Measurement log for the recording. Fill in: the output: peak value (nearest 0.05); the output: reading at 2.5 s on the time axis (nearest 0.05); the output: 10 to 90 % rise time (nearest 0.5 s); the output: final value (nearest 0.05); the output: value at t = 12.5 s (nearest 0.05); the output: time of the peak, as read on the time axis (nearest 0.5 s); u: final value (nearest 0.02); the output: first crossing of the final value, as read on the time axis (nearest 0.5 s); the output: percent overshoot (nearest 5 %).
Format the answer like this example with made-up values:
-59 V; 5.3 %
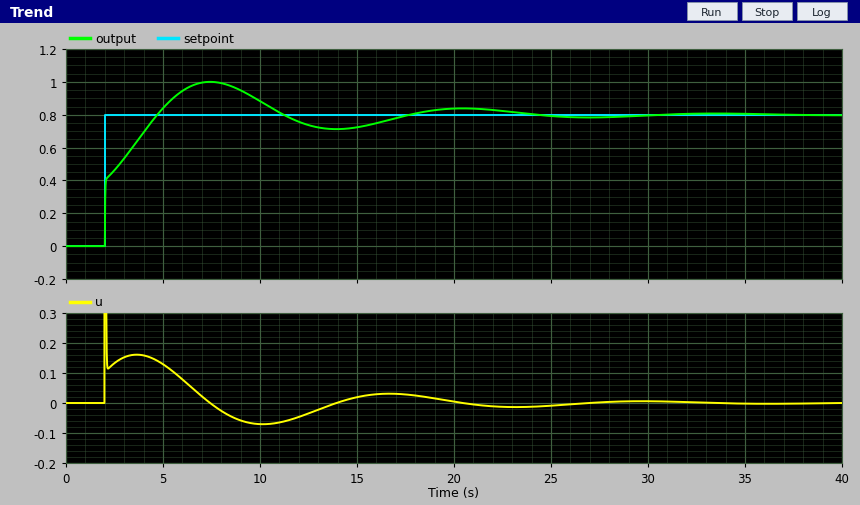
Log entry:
1.00; 0.45; 2.0 s; 0.80; 0.75; 7.5 s; 0.00; 4.5 s; 25 %
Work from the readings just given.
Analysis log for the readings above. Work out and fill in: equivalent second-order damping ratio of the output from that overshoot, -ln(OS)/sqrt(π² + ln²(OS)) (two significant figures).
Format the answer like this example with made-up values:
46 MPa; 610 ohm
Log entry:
0.40
